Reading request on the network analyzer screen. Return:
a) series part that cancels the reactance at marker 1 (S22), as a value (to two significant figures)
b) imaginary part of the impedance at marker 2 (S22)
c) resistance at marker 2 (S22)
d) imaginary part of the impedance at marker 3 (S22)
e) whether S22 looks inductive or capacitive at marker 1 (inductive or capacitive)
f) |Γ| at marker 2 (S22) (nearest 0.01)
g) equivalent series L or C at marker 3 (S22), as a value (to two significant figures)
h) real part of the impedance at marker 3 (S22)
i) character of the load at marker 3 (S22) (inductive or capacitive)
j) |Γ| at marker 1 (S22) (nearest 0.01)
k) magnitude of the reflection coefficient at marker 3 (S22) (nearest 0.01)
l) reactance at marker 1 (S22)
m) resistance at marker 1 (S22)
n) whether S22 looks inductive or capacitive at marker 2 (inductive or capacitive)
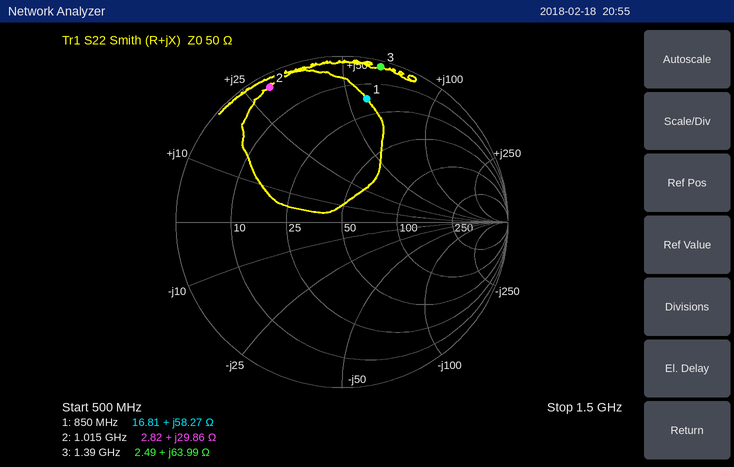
3.2 pF
+29.86 Ω
2.82 Ω
+63.99 Ω
inductive
0.92
7.3 nH
2.49 Ω
inductive
0.76
0.96
+58.27 Ω
16.81 Ω
inductive
